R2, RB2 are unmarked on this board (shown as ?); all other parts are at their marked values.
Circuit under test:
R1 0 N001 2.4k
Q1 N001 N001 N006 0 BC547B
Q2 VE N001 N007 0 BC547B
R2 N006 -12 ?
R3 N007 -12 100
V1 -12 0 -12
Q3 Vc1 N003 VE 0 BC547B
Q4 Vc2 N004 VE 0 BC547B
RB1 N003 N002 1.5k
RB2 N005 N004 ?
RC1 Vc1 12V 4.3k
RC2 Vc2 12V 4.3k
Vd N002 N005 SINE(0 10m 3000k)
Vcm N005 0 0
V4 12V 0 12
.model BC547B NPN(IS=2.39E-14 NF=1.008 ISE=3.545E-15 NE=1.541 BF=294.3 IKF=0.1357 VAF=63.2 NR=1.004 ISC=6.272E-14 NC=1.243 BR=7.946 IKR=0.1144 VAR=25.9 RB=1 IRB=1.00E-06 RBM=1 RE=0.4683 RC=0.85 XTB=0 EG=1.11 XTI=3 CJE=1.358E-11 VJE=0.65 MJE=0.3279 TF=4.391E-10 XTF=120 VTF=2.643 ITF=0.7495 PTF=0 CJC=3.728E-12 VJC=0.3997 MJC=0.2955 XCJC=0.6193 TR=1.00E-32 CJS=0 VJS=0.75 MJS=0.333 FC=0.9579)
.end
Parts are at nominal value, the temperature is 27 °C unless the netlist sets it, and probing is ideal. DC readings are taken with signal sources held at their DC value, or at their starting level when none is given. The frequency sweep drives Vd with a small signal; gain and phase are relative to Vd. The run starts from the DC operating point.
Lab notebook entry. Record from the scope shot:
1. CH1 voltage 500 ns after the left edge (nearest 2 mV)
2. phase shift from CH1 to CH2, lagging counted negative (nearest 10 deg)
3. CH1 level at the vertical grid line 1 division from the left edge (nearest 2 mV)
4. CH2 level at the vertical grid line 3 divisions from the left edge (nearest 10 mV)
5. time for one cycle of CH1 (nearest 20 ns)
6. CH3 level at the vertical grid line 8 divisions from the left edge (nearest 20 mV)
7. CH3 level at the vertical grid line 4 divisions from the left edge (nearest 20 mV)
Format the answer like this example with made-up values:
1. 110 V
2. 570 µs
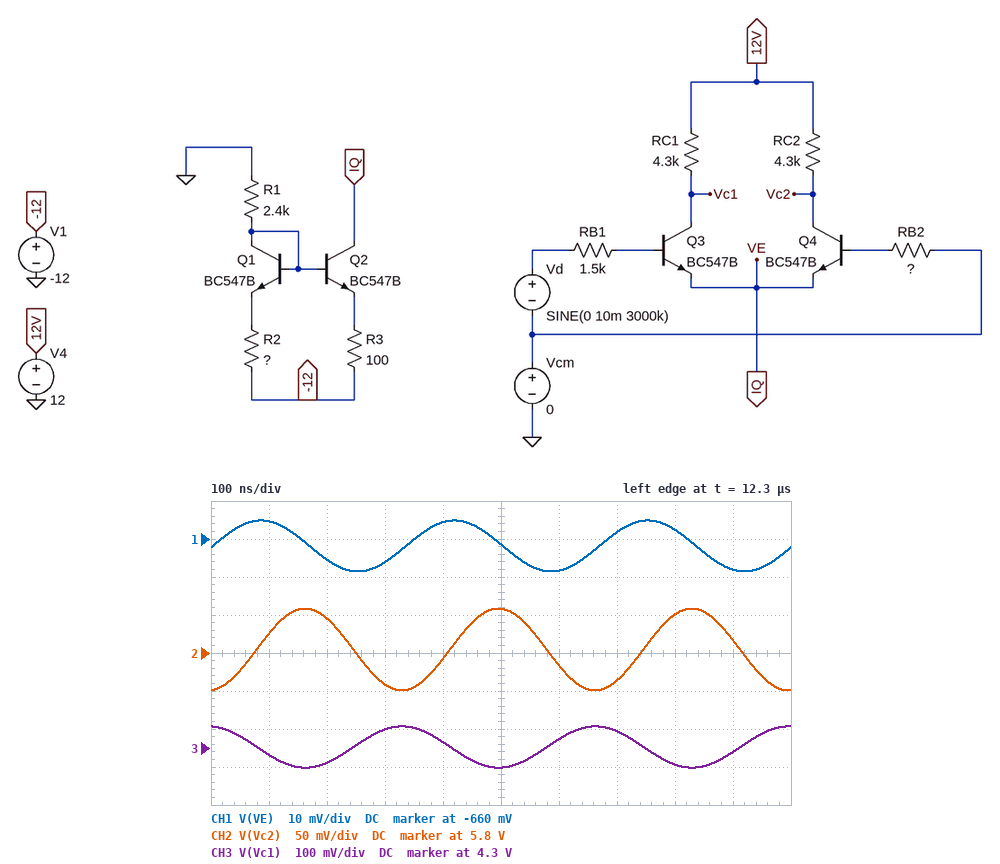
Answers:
1. -662 mV
2. -80 deg
3. -656 mV
4. 5.76 V
5. 340 ns
6. 4.26 V
7. 4.32 V
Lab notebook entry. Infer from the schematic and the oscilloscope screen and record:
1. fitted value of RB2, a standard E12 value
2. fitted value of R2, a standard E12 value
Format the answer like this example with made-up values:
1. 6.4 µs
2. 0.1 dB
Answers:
1. 3.3 kΩ
2. 68 Ω
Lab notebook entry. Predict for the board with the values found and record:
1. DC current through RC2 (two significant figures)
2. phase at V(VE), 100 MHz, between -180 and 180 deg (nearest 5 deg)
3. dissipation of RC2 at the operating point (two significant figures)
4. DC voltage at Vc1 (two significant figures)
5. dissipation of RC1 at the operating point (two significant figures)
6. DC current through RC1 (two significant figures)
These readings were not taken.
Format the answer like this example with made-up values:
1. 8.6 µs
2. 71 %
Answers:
1. 1.4 mA
2. -40 deg
3. 8.9 mW
4. 4.3 V
5. 14 mW
6. 1.8 mA
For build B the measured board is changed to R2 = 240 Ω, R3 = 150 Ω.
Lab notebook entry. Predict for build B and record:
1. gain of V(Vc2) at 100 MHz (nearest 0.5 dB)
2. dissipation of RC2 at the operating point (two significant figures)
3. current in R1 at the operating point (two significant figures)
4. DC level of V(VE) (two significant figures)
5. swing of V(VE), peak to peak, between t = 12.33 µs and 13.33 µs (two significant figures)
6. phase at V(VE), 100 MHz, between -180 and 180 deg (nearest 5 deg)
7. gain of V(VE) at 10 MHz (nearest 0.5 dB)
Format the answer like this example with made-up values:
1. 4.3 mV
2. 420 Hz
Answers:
1. -12.0 dB
2. 41 mW
3. 4.3 mA
4. -1.3 V
5. 9.2 mV
6. -30 deg
7. -7.0 dB
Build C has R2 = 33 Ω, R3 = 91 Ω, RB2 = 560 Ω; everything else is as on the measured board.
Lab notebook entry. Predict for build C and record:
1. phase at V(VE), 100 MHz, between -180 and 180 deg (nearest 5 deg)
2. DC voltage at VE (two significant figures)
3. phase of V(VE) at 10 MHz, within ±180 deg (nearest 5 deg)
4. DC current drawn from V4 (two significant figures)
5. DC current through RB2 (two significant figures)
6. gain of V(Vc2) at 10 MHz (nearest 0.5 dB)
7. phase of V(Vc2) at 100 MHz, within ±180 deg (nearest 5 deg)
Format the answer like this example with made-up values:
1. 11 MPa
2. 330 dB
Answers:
1. -25 deg
2. -640 mV
3. -5 deg
4. 2.0 mA
5. 3.3 µA
6. 11.5 dB
7. -100 deg
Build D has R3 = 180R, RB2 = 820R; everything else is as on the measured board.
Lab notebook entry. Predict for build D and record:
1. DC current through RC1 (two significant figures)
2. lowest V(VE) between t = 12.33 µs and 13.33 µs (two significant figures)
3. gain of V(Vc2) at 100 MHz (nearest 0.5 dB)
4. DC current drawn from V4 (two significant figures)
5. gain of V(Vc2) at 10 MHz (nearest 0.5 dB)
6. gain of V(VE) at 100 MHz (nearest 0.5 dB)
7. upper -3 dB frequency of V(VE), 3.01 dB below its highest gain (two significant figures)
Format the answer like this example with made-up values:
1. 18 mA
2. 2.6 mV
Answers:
1. 910 µA
2. -640 mV
3. -16.5 dB
4. 1.9 mA
5. 10.5 dB
6. -12.5 dB
7. 24 MHz
